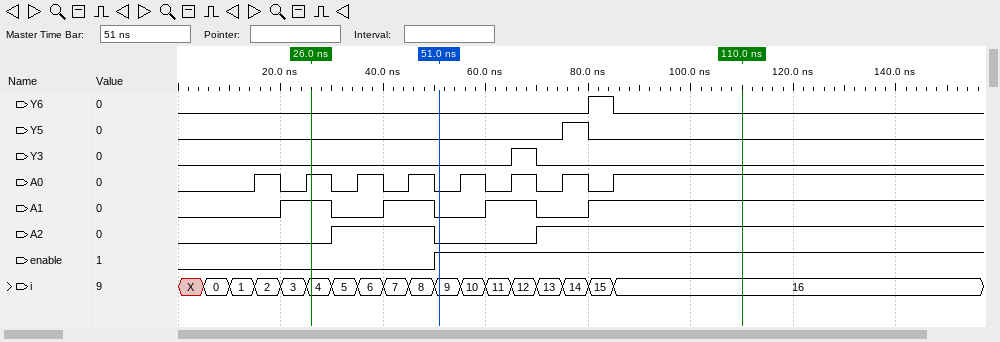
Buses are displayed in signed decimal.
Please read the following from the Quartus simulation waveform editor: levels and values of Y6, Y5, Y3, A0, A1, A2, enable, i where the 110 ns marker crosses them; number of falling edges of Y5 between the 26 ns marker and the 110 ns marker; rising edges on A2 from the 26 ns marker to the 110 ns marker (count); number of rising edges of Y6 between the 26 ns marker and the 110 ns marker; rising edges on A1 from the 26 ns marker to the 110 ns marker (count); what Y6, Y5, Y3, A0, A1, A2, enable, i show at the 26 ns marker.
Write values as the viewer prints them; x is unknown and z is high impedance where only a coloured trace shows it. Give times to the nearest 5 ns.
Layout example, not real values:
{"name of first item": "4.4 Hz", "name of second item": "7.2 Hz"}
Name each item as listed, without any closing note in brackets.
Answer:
{"levels and values of Y6, Y5, Y3, A0, A1, A2, enable, i where the 110 ns marker crosses them": "Y6=0, Y5=0, Y3=0, A0=1, A1=1, A2=1, enable=1, i=16", "number of falling edges of Y5 between the 26 ns marker and the 110 ns marker": "1", "rising edges on A2 from the 26 ns marker to the 110 ns marker": "2", "number of rising edges of Y6 between the 26 ns marker and the 110 ns marker": "1", "rising edges on A1 from the 26 ns marker to the 110 ns marker": "3", "what Y6, Y5, Y3, A0, A1, A2, enable, i show at the 26 ns marker": "Y6=0, Y5=0, Y3=0, A0=1, A1=1, A2=0, enable=0, i=4"}
